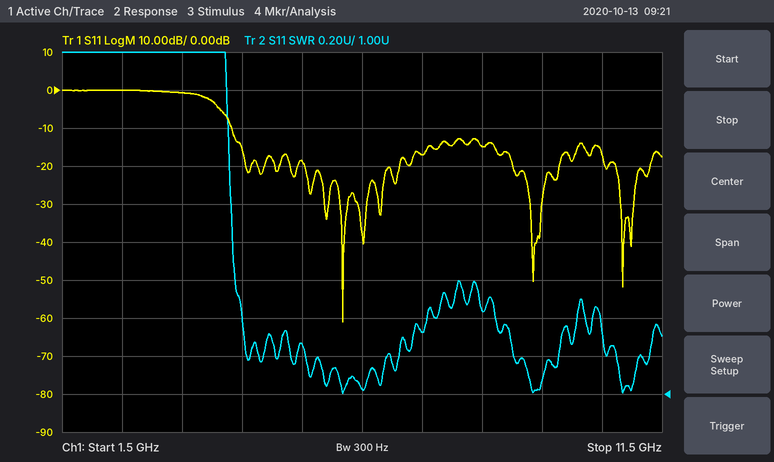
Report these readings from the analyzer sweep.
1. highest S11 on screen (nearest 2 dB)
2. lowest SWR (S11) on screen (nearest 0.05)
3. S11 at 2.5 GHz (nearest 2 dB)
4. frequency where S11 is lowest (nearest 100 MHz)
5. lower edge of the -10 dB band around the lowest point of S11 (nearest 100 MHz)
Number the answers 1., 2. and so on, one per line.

1. 0 dB
2. 1.00
3. 0 dB
4. 6.2 GHz
5. 4.3 GHz
